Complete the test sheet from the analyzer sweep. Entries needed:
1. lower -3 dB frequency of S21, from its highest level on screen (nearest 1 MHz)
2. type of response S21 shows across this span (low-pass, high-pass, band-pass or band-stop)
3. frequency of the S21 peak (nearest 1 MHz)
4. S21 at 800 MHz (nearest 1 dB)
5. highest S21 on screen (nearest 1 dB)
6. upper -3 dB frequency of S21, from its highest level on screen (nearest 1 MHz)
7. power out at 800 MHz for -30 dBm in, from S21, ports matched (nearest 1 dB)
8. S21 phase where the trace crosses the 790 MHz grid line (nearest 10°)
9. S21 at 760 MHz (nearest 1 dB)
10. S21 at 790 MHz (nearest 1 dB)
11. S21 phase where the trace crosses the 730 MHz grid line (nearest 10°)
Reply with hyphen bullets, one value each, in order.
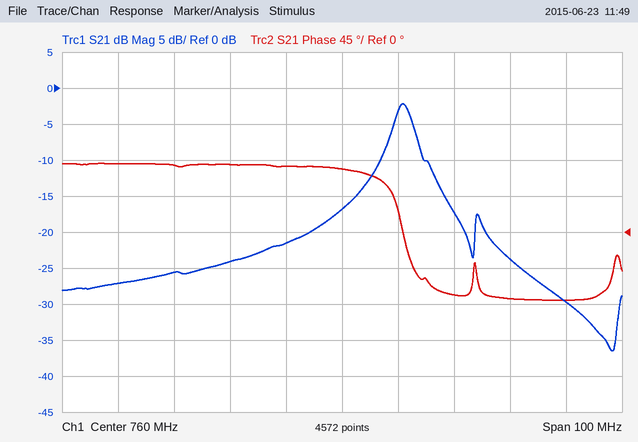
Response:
- 769 MHz
- band-pass
- 771 MHz
- -30 dB
- -2 dB
- 773 MHz
- -60 dBm
- -80°
- -17 dB
- -24 dB
- 80°
